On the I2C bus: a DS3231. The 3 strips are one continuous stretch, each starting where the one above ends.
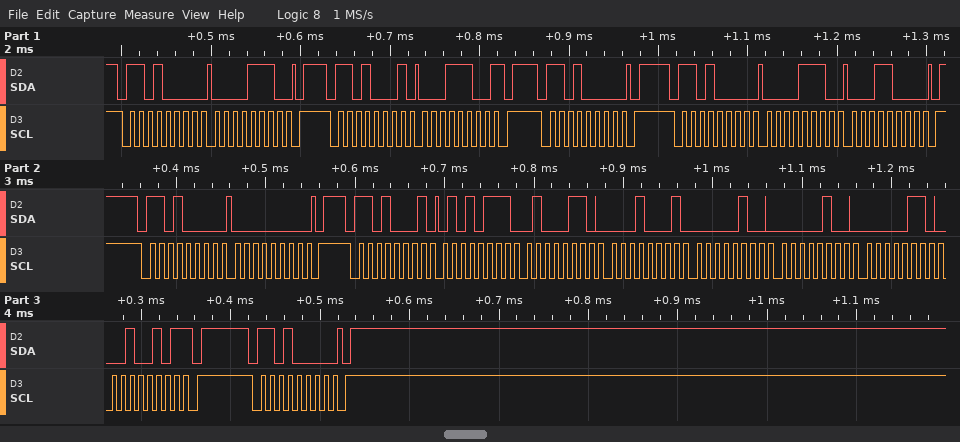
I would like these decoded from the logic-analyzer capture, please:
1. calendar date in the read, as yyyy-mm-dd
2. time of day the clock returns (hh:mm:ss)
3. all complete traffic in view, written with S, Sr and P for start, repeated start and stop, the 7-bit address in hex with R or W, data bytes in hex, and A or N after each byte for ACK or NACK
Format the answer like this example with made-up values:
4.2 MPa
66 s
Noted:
2025-06-04
11:46:57
S 68W A 0E A P S 68R A 1C N P S 68W A P S 68W A 0E A 18 A P S 68W A 00 A P S 68R A 57 A 46 A 11 A 04 A 04 A 06 A 25 N P S 68W A P
